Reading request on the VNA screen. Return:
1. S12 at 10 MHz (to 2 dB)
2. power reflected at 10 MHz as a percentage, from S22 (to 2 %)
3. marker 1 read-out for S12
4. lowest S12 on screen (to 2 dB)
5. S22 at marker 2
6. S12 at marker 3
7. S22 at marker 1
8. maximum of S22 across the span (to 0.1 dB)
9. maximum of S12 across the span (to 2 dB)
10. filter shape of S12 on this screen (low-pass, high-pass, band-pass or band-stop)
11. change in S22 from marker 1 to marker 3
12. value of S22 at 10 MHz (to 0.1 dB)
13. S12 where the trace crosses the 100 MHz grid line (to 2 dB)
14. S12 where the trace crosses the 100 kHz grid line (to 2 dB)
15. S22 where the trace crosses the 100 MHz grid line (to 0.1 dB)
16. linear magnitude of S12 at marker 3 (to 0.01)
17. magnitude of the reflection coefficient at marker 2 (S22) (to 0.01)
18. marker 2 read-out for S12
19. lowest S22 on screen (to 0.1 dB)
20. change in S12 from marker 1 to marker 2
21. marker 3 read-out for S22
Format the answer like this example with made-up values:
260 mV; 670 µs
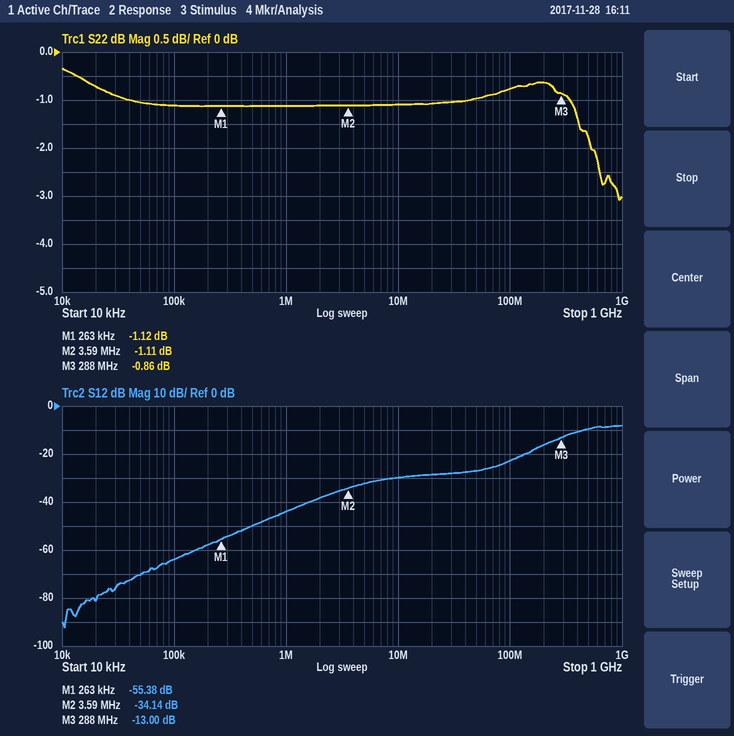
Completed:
-30 dB; 78 %; -55.38 dB; -92 dB; -1.11 dB; -13.00 dB; -1.12 dB; -0.3 dB; -8 dB; high-pass; 0.26 dB; -1.1 dB; -22 dB; -64 dB; -0.8 dB; 0.22; 0.88; -34.14 dB; -3.1 dB; 21.24 dB; -0.86 dB
